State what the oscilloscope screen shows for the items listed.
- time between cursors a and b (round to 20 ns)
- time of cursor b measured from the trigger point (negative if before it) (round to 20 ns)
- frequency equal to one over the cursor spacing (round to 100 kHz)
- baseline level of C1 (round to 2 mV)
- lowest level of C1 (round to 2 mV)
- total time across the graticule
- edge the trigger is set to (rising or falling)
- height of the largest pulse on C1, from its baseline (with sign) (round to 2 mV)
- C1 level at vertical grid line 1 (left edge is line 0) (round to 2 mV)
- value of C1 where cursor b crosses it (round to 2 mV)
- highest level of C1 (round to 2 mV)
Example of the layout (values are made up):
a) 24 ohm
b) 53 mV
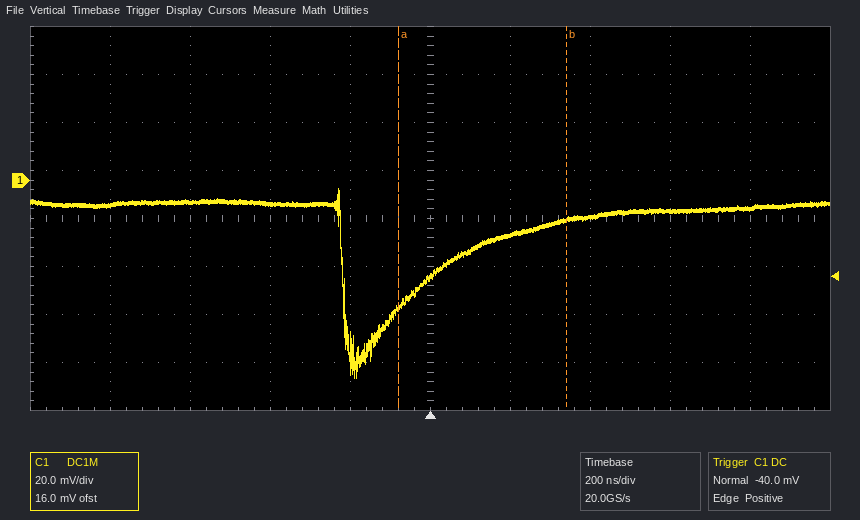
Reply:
a) 420 ns
b) +340 ns
c) 2.4 MHz
d) -10 mV
e) -82 mV
f) 2 µs
g) rising
h) -72 mV
i) -10 mV
j) -16 mV
k) -4 mV
